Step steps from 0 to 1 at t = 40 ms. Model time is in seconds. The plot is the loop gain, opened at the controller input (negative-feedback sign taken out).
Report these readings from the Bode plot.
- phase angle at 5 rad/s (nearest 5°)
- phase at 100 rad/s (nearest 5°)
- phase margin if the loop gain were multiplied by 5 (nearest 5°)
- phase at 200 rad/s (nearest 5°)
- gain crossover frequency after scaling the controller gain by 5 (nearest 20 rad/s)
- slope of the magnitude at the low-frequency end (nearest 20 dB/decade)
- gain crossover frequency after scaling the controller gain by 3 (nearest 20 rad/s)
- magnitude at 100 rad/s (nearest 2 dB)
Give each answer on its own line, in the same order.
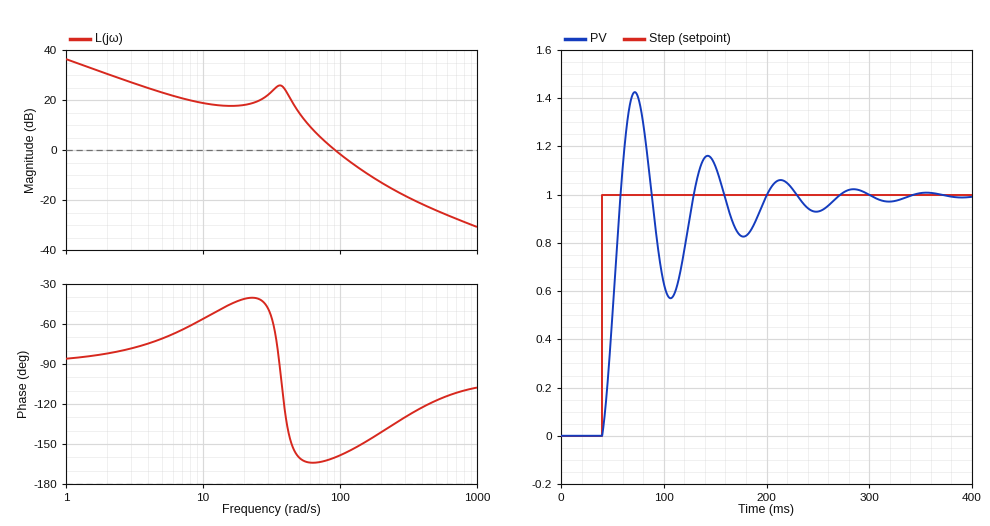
-70°
-160°
40°
-140°
220 rad/s
-20 dB/decade
160 rad/s
-2 dB
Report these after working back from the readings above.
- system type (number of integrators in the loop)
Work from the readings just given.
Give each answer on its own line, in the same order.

1
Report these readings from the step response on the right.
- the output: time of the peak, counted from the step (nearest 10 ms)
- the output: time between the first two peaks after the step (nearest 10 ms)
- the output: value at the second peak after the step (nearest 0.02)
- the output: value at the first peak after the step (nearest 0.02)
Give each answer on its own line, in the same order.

30 ms
70 ms
1.16
1.42
